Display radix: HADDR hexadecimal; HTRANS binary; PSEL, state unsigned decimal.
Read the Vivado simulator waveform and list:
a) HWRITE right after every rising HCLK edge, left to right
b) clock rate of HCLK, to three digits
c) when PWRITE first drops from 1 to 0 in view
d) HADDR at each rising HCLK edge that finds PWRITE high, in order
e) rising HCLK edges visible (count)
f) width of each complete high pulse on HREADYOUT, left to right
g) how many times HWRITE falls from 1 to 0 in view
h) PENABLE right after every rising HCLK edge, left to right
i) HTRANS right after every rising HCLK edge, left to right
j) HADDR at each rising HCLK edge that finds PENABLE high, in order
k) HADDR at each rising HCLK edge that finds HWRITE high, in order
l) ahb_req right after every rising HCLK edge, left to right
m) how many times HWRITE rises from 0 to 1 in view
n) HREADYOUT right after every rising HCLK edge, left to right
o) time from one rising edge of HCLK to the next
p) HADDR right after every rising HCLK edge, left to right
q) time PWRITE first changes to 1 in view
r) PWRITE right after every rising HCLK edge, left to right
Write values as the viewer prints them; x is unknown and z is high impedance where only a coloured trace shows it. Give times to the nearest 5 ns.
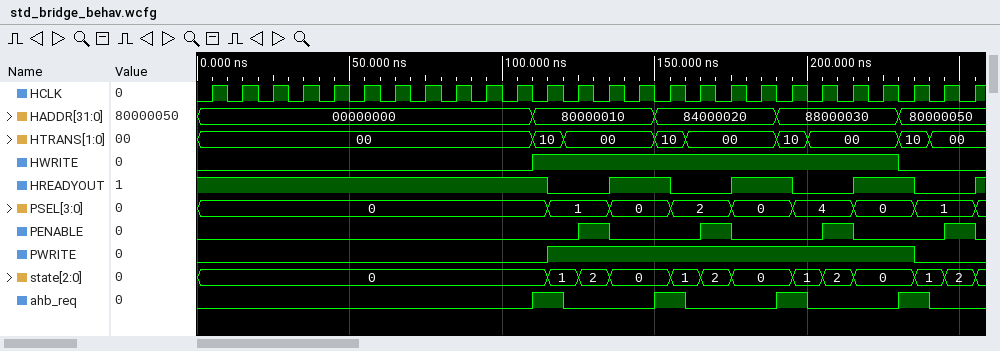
0 0 0 0 0 0 0 0 0 0 0 1 1 1 1 1 1 1 1 1 1 1 1 0 0 0
100 MHz
235 ns
80000010, 80000010, 80000010, 84000020, 84000020, 84000020, 84000020, 88000030, 88000030, 88000030, 88000030, 80000050
26
20 ns, 20 ns, 20 ns
1
0 0 0 0 0 0 0 0 0 0 0 0 1 0 0 0 1 0 0 0 1 0 0 0 1 0
00, 00, 00, 00, 00, 00, 00, 00, 00, 00, 00, 10, 00, 00, 00, 10, 00, 00, 00, 10, 00, 00, 00, 10, 00, 00
80000010, 84000020, 88000030, 80000050
80000010, 80000010, 80000010, 80000010, 84000020, 84000020, 84000020, 84000020, 88000030, 88000030, 88000030, 88000030
0 0 0 0 0 0 0 0 0 0 0 1 0 0 0 1 0 0 0 1 0 0 0 1 0 0
1
1 1 1 1 1 1 1 1 1 1 1 0 0 1 1 0 0 1 1 0 0 1 1 0 0 1
10 ns
00000000, 00000000, 00000000, 00000000, 00000000, 00000000, 00000000, 00000000, 00000000, 00000000, 00000000, 80000010, 80000010, 80000010, 80000010, 84000020, 84000020, 84000020, 84000020, 88000030, 88000030, 88000030, 88000030, 80000050, 80000050, 80000050
115 ns
0 0 0 0 0 0 0 0 0 0 0 1 1 1 1 1 1 1 1 1 1 1 1 0 0 0
